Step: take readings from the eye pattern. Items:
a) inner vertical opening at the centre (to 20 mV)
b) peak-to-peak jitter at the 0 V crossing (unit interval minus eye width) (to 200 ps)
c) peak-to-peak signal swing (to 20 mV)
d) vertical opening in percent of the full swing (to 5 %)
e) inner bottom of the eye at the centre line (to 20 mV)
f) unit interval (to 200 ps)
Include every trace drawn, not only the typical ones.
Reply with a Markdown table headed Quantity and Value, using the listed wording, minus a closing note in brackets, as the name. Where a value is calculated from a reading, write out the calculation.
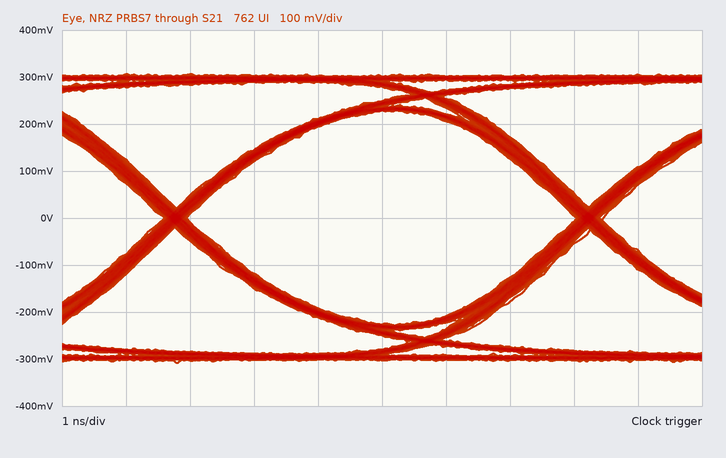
| Quantity | Value |
|---|---|
| inner vertical opening at the centre | 460 mV |
| peak-to-peak jitter at the 0 V crossing (unit interval minus eye width) | 400 ps |
| peak-to-peak signal swing | 620 mV |
| vertical opening in percent of the full swing | 460 mV / 620 mV ≈ 74.2 %, so 75 % to the nearest 5 % |
| inner bottom of the eye at the centre line | -220 mV |
| unit interval | 6.4 ns |
